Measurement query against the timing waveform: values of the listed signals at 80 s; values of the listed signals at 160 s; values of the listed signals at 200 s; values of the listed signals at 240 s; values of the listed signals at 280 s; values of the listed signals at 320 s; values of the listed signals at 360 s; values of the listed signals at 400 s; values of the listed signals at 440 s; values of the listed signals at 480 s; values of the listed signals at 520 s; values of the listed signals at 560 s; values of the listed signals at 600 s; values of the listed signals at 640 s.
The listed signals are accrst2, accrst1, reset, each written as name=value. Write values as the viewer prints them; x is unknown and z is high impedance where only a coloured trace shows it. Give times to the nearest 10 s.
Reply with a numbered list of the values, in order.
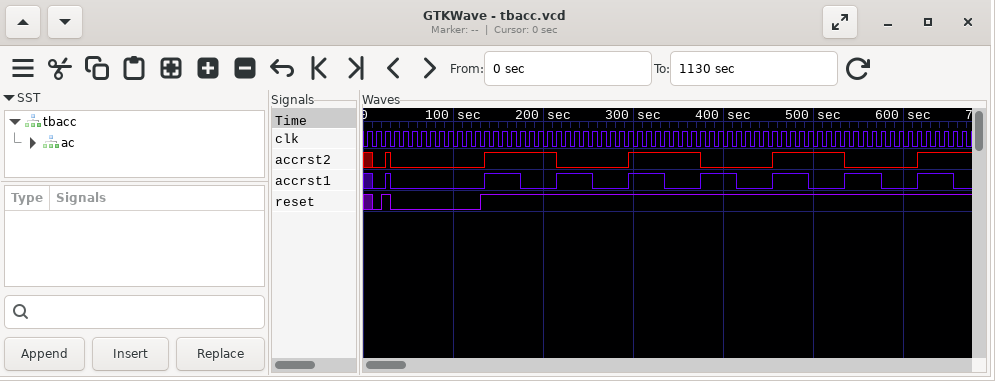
1. accrst2=0, accrst1=0, reset=0
2. accrst2=1, accrst1=1, reset=1
3. accrst2=1, accrst1=0, reset=1
4. accrst2=0, accrst1=1, reset=1
5. accrst2=0, accrst1=0, reset=1
6. accrst2=1, accrst1=1, reset=1
7. accrst2=1, accrst1=0, reset=1
8. accrst2=0, accrst1=1, reset=1
9. accrst2=0, accrst1=0, reset=1
10. accrst2=1, accrst1=1, reset=1
11. accrst2=1, accrst1=0, reset=1
12. accrst2=0, accrst1=1, reset=1
13. accrst2=0, accrst1=0, reset=1
14. accrst2=1, accrst1=1, reset=1
